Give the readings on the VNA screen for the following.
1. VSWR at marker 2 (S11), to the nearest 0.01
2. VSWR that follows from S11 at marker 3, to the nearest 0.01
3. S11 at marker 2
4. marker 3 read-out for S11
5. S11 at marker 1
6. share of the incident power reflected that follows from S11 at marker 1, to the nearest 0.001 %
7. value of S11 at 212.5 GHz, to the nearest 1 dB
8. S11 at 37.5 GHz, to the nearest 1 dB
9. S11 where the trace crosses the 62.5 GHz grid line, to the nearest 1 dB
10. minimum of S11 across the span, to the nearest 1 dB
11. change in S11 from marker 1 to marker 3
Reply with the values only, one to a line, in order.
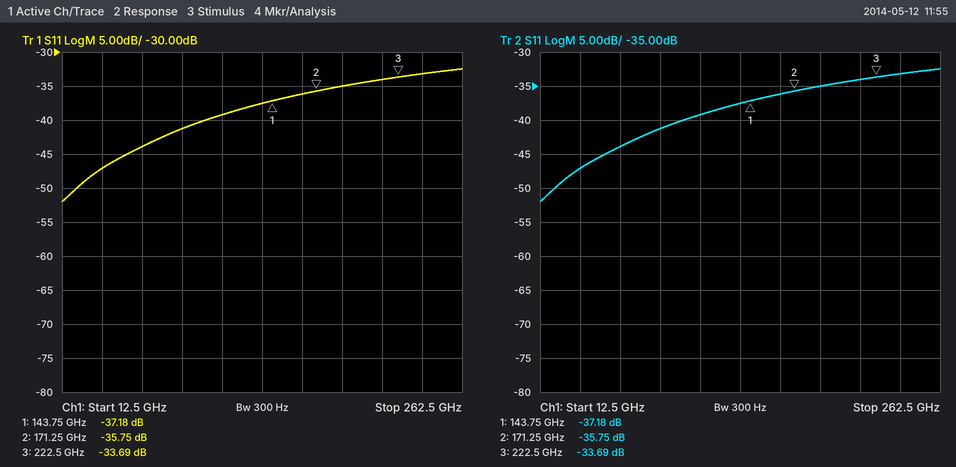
1.03
1.04
-35.75 dB
-33.69 dB
-37.18 dB
0.019 %
-34 dB
-47 dB
-44 dB
-52 dB
3.49 dB
